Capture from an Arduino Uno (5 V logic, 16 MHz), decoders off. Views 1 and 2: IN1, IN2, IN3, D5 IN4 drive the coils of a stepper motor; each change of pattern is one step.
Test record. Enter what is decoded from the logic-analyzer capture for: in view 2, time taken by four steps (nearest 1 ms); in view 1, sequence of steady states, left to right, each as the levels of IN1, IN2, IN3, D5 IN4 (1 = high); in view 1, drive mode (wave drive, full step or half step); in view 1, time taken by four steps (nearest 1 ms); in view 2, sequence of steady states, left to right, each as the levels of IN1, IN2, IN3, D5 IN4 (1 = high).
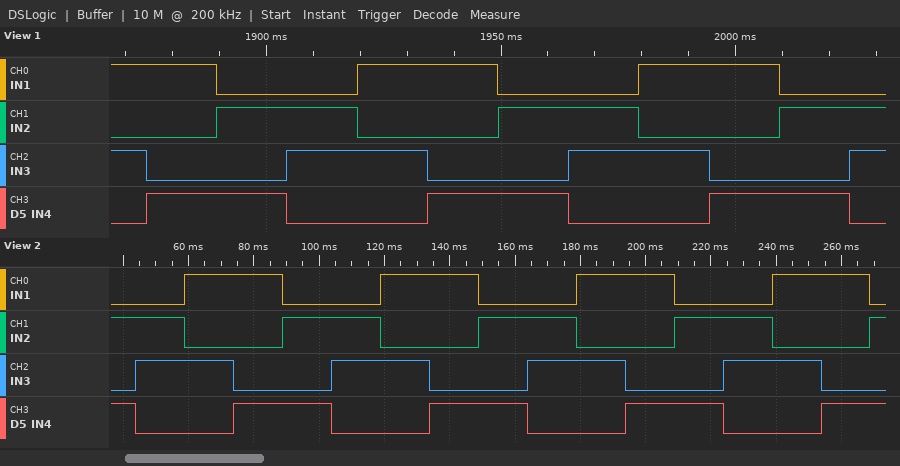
60 ms
1010 1001 0101 0110 1010 1001 0101 0110 1010 1001 0101 0110
full step
60 ms
0101 0110 1010 1001 0101 0110 1010 1001 0101 0110 1010 1001 0101 0110 1010 1001 0101
